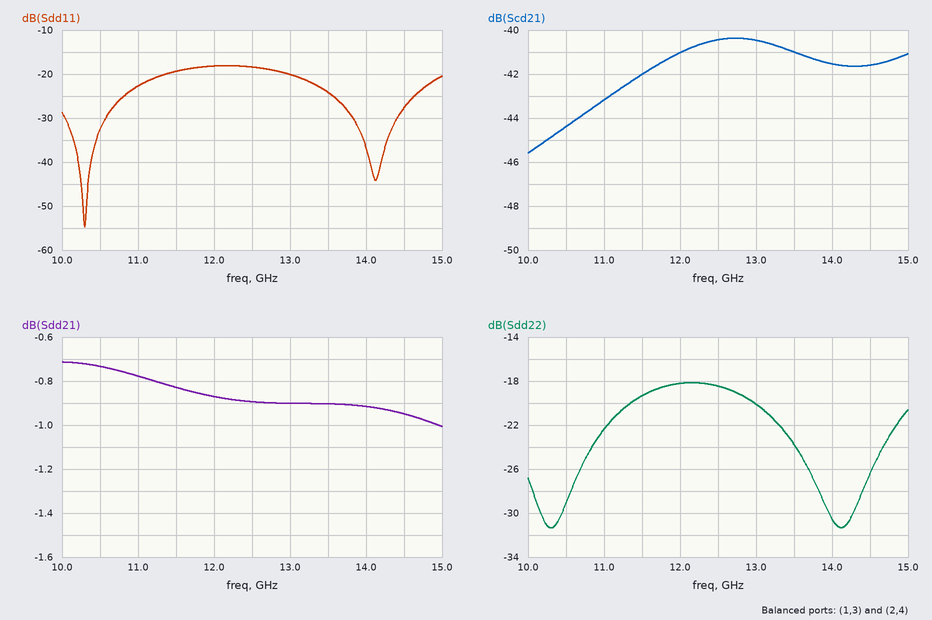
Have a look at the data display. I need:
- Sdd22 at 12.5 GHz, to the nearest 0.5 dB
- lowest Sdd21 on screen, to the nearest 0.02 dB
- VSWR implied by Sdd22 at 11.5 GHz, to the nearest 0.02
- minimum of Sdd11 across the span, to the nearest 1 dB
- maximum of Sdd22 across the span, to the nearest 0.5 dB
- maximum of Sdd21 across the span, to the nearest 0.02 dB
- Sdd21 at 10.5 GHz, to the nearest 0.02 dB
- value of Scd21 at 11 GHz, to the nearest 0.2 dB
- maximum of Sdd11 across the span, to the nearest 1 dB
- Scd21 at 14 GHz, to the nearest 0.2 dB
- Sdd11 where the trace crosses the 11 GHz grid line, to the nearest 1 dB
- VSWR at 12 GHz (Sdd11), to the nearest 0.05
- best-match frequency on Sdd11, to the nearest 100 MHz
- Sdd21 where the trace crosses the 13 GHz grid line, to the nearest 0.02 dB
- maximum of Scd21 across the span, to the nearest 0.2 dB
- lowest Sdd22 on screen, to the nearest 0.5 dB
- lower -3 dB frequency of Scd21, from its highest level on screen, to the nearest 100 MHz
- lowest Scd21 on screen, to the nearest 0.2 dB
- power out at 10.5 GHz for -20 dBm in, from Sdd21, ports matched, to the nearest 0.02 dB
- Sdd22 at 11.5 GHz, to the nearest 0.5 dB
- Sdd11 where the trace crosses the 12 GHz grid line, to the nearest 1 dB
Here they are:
-18.5 dB
-1.00 dB
1.24
-55 dB
-18.0 dB
-0.72 dB
-0.74 dB
-43.2 dB
-18 dB
-41.6 dB
-23 dB
1.30
10.3 GHz
-0.90 dB
-40.4 dB
-31.5 dB
10.9 GHz
-45.6 dB
-20.74 dBm
-19.5 dB
-18 dB
